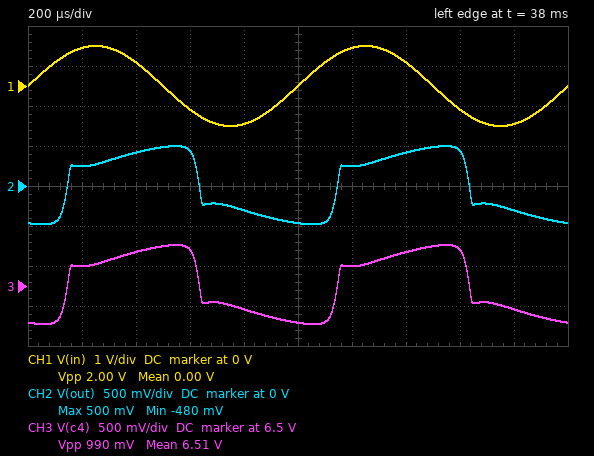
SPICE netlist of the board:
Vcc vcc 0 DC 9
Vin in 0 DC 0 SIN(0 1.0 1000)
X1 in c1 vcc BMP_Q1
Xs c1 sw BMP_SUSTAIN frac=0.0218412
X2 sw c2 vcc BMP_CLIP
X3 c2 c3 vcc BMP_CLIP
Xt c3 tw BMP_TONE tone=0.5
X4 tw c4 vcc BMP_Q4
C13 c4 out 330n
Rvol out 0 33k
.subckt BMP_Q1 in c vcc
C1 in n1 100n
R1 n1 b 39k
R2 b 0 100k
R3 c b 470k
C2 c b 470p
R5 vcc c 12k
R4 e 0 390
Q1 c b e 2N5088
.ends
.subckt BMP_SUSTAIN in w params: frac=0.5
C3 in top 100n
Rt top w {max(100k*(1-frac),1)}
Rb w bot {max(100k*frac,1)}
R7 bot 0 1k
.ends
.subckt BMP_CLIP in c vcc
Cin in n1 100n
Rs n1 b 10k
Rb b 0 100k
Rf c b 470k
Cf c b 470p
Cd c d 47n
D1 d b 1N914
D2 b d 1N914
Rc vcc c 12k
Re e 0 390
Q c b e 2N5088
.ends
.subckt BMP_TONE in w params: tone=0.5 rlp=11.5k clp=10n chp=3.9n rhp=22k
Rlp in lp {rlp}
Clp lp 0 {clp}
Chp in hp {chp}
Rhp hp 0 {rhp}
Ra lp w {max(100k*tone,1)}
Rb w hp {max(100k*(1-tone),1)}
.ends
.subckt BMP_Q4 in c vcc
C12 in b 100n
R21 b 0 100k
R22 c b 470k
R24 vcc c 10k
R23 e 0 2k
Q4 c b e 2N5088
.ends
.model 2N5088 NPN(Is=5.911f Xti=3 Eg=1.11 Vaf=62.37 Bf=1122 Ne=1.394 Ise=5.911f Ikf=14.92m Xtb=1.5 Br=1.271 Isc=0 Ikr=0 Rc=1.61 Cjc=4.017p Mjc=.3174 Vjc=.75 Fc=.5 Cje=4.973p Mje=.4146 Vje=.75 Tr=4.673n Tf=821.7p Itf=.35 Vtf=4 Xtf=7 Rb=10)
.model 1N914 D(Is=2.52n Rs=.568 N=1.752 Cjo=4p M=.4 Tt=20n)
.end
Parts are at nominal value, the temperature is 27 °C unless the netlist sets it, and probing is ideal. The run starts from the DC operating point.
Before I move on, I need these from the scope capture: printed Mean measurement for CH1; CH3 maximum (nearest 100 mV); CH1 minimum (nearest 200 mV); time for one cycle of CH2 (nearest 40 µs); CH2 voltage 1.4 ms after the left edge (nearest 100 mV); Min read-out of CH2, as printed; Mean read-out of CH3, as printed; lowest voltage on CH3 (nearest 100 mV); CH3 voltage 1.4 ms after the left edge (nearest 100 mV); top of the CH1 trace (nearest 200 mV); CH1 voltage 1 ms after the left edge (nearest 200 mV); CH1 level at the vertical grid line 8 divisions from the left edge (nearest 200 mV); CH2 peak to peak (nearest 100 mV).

0.00 V
7.0 V
-1.0 V
1.00 ms
400 mV
-480 mV
6.51 V
6.0 V
6.9 V
1.0 V
0 V
-600 mV
1.0 V
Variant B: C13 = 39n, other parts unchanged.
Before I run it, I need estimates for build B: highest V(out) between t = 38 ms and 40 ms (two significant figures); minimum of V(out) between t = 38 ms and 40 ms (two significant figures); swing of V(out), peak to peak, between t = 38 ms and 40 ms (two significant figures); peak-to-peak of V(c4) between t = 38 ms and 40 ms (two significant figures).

470 mV
-450 mV
920 mV
1.0 V
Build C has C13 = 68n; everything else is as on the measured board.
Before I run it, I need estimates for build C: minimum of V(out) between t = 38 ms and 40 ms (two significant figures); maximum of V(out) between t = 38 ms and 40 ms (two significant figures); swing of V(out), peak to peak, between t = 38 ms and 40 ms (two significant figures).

-470 mV
480 mV
950 mV
